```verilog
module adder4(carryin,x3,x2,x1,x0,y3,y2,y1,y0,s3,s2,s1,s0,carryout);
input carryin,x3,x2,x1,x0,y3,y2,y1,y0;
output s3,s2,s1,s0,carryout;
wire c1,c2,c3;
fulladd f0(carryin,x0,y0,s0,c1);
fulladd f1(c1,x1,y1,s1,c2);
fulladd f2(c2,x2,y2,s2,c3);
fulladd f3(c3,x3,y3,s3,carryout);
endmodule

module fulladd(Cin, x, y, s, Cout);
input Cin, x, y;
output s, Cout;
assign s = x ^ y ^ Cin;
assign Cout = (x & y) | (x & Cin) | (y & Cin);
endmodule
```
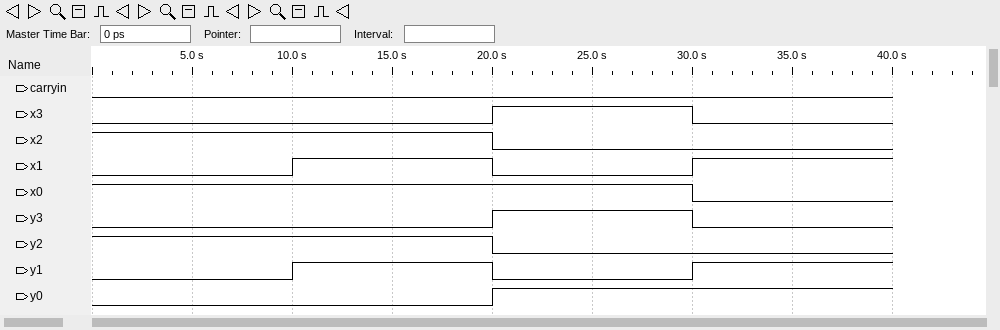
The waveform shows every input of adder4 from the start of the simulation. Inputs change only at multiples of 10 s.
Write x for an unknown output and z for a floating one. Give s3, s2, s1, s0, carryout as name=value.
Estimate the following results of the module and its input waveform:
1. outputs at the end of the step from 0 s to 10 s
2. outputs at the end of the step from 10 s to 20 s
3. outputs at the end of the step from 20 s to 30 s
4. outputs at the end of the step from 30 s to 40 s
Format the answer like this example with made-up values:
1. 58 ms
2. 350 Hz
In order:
1. s3=1, s2=0, s1=0, s0=1, carryout=0
2. s3=1, s2=1, s1=0, s0=1, carryout=0
3. s3=0, s2=0, s1=1, s0=0, carryout=1
4. s3=0, s2=1, s1=0, s0=1, carryout=0
